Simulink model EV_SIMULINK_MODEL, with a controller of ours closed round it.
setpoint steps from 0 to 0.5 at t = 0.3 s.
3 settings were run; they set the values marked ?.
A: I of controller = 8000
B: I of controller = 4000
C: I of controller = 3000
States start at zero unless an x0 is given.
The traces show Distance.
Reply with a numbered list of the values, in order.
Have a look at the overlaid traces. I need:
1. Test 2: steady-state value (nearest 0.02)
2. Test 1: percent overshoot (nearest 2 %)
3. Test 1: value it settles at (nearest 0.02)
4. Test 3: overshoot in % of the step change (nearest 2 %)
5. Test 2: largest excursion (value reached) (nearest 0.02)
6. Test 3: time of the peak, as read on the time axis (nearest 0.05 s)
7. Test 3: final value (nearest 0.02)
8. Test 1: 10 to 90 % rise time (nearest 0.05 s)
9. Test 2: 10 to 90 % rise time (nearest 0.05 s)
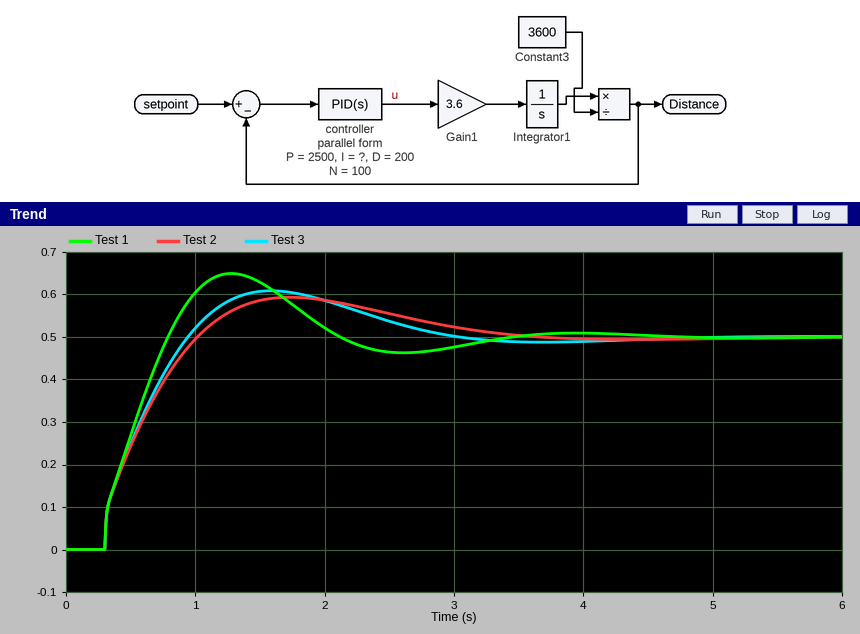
1. 0.50
2. 30 %
3. 0.50
4. 22 %
5. 0.60
6. 1.60 s
7. 0.50
8. 0.40 s
9. 0.55 s
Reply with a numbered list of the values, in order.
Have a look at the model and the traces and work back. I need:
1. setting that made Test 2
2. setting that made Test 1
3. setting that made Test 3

1. C
2. A
3. B
